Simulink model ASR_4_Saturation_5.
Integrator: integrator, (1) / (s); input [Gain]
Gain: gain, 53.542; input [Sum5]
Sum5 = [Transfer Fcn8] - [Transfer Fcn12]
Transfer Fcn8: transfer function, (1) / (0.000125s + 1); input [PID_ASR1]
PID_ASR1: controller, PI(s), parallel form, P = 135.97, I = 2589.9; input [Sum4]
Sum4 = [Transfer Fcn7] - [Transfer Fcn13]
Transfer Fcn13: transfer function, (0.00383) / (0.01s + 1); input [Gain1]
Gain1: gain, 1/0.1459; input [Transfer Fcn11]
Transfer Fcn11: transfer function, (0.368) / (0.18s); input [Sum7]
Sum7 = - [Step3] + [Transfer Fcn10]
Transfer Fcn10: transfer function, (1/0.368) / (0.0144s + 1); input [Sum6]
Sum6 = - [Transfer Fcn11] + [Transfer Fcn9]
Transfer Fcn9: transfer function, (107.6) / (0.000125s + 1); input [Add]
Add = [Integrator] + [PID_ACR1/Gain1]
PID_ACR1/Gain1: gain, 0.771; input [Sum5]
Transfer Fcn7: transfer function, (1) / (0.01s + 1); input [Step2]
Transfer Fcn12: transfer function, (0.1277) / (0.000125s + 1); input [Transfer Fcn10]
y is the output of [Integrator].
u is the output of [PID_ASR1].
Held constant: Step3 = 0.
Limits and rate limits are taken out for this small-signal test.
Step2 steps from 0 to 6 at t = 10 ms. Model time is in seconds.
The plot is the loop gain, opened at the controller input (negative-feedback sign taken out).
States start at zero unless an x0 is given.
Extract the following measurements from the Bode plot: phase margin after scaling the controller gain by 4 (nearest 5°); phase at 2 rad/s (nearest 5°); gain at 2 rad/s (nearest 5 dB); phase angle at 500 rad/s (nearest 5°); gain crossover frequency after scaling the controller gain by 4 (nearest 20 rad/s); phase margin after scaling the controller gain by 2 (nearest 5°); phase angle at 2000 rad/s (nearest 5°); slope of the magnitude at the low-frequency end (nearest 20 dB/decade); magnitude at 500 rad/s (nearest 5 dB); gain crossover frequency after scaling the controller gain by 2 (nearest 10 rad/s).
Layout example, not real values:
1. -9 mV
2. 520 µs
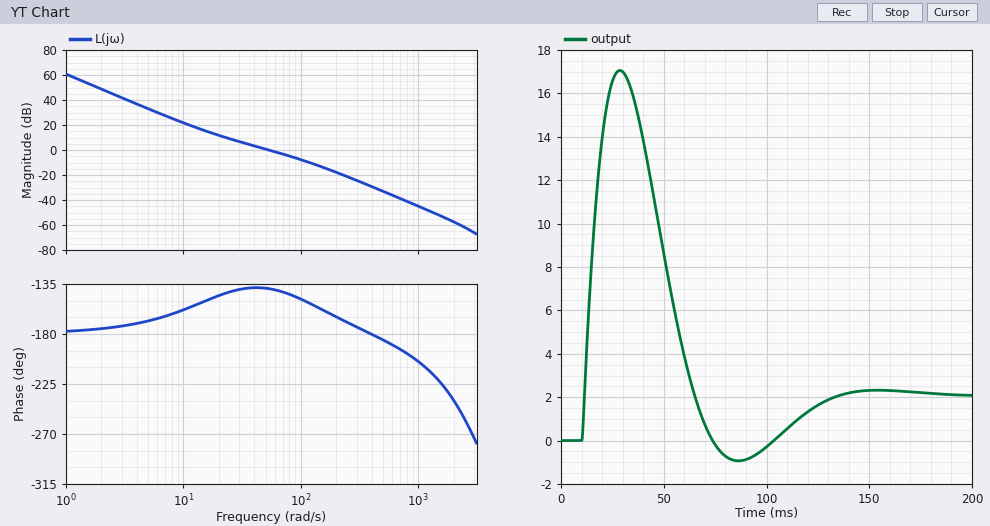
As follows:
1. 25°
2. -175°
3. 50 dB
4. -185°
5. 140 rad/s
6. 35°
7. -240°
8. -40 dB/decade
9. -35 dB
10. 90 rad/s
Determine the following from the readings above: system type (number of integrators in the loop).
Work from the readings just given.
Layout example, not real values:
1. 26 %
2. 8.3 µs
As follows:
1. 2
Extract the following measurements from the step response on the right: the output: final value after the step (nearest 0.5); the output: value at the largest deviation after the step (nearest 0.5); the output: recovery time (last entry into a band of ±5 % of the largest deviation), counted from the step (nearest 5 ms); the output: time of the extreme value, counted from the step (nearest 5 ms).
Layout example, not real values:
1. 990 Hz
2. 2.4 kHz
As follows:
1. 2.0
2. 17.0
3. 110 ms
4. 20 ms
